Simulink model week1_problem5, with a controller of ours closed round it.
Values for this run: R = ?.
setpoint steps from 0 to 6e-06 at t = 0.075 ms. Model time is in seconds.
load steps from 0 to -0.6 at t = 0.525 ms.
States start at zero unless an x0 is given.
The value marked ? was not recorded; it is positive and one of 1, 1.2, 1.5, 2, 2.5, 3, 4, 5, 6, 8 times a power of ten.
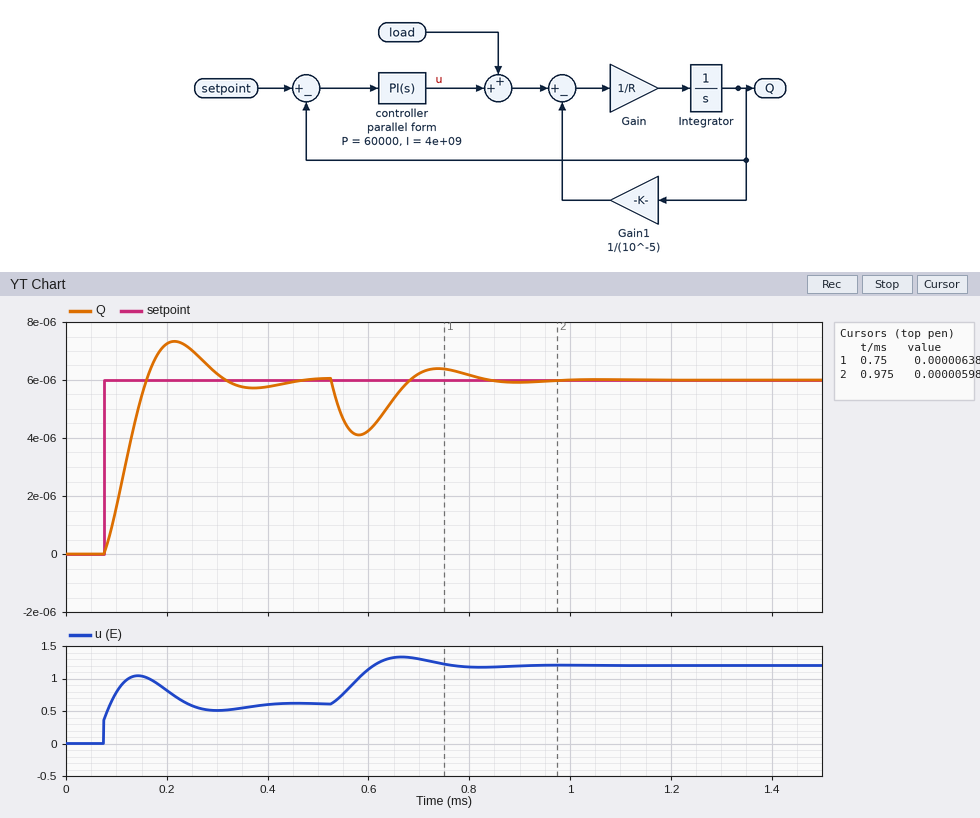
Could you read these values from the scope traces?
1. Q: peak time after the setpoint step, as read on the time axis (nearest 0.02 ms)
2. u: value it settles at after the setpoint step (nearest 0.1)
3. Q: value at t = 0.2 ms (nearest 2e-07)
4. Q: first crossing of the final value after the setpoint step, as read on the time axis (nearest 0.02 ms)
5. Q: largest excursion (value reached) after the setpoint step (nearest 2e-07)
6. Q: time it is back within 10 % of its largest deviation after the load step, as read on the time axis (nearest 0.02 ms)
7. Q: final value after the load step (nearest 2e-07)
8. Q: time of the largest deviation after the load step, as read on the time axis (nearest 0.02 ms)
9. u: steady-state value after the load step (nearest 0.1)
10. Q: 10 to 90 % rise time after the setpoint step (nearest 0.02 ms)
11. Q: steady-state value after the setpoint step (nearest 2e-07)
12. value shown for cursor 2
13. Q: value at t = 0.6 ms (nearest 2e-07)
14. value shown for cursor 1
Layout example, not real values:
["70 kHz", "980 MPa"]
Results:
["0.22 ms", "0.6", "0.0000072", "0.16 ms", "0.0000074", "0.80 ms", "0.0000060", "0.58 ms", "1.2", "0.06 ms", "0.0000060", "0.00000598", "0.0000042", "0.00000638"]
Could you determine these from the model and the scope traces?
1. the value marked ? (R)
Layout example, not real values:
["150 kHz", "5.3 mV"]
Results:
["8"]
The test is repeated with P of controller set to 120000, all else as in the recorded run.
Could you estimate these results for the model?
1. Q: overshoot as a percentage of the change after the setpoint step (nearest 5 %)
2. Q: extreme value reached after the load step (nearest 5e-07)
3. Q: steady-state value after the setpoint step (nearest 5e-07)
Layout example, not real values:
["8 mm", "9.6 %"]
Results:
["10 %", "0.0000045", "0.0000060"]
